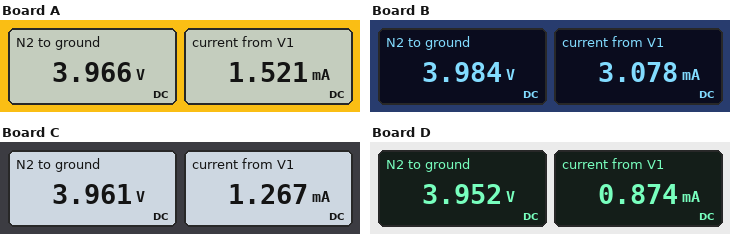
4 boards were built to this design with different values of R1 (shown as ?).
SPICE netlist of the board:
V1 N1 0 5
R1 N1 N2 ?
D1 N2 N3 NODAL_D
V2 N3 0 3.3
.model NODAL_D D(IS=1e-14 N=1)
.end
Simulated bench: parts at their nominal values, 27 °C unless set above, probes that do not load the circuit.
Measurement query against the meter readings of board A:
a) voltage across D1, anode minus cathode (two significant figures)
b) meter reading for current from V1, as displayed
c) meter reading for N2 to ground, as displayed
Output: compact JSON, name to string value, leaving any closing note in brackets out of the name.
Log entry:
{"voltage across D1, anode minus cathode": "670 mV", "meter reading for current from V1, as displayed": "1.521 mA", "meter reading for N2 to ground, as displayed": "3.966 V"}
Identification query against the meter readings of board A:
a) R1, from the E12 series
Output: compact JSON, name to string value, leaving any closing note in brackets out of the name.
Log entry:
{"R1, from the E12 series": "680 Ω"}
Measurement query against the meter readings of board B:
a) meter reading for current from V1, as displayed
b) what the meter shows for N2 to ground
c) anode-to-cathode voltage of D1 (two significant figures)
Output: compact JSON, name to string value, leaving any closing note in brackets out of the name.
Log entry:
{"meter reading for current from V1, as displayed": "3.078 mA", "what the meter shows for N2 to ground": "3.984 V", "anode-to-cathode voltage of D1": "680 mV"}
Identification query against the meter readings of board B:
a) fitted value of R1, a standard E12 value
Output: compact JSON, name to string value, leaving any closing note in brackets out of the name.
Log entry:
{"fitted value of R1, a standard E12 value": "330 Ω"}
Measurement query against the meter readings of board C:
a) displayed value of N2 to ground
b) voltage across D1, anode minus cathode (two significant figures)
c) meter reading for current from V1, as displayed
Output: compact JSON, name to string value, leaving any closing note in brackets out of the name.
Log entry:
{"displayed value of N2 to ground": "3.961 V", "voltage across D1, anode minus cathode": "660 mV", "meter reading for current from V1, as displayed": "1.267 mA"}
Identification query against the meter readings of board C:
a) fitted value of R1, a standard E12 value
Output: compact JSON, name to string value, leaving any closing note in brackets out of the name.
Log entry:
{"fitted value of R1, a standard E12 value": "820 Ω"}
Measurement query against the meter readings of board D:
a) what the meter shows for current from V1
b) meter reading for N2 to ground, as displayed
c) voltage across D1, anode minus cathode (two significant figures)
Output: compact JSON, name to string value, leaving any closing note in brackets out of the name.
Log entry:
{"what the meter shows for current from V1": "0.874 mA", "meter reading for N2 to ground, as displayed": "3.952 V", "voltage across D1, anode minus cathode": "650 mV"}
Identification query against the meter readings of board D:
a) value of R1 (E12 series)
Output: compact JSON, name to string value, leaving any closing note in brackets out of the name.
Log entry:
{"value of R1": "1.2 kΩ"}
